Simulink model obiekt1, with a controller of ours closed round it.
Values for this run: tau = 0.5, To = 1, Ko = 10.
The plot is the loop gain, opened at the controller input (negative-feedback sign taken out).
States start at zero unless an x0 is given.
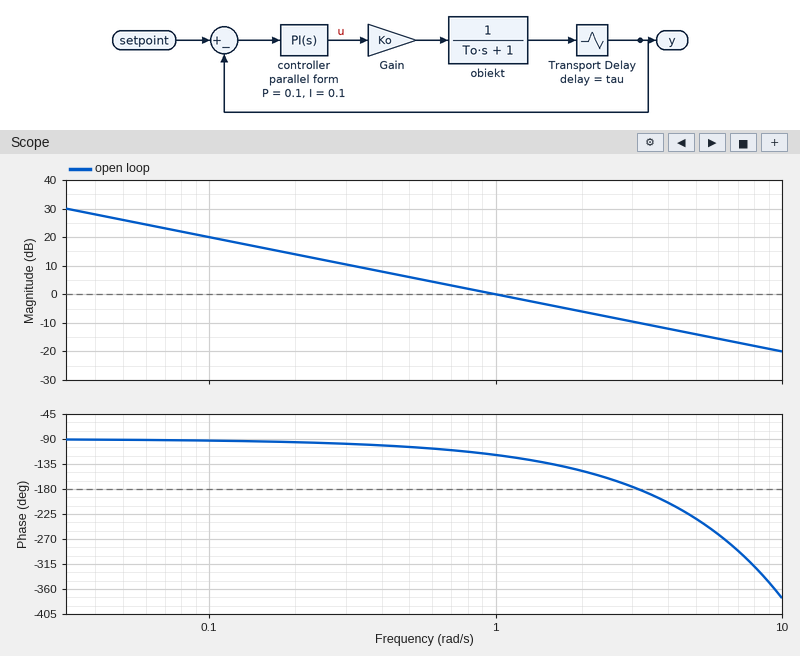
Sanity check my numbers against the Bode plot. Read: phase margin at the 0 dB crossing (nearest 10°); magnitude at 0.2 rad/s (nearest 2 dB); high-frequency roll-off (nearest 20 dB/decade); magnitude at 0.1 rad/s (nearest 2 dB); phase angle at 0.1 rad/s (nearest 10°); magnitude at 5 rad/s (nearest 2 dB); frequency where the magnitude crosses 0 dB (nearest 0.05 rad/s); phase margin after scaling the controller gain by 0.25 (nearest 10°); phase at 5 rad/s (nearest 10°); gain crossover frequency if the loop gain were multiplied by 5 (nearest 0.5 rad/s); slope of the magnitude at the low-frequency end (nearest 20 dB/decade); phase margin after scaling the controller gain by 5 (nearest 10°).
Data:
60°
14 dB
-20 dB/decade
20 dB
-90°
-14 dB
1.00 rad/s
80°
-230°
5.0 rad/s
-20 dB/decade
-50°
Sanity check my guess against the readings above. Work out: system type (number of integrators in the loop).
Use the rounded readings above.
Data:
1
